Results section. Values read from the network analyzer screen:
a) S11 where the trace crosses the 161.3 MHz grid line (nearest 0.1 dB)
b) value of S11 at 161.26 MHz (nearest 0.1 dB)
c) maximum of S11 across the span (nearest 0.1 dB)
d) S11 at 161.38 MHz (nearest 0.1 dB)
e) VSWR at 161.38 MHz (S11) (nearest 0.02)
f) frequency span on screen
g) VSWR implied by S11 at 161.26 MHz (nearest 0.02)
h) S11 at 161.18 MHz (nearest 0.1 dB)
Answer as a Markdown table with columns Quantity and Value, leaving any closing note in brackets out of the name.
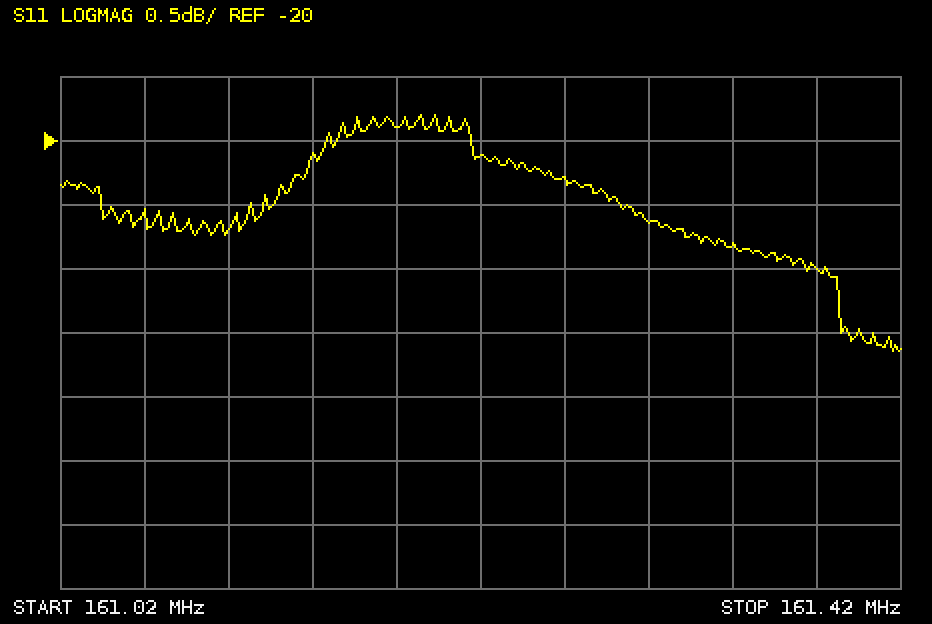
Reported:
| Quantity | Value |
|---|---|
| S11 where the trace crosses the 161.3 MHz grid line | -20.6 dB |
| value of S11 at 161.26 MHz | -20.3 dB |
| maximum of S11 across the span | -19.8 dB |
| S11 at 161.38 MHz | -21.0 dB |
| VSWR at 161.38 MHz (S11) | 1.20 |
| frequency span on screen | 400 kHz |
| VSWR implied by S11 at 161.26 MHz | 1.22 |
| S11 at 161.18 MHz | -19.9 dB |
